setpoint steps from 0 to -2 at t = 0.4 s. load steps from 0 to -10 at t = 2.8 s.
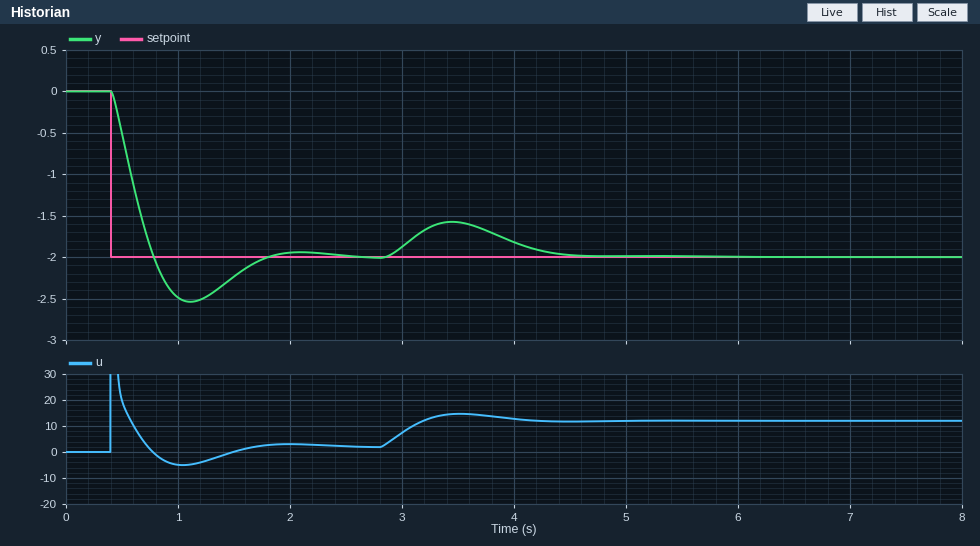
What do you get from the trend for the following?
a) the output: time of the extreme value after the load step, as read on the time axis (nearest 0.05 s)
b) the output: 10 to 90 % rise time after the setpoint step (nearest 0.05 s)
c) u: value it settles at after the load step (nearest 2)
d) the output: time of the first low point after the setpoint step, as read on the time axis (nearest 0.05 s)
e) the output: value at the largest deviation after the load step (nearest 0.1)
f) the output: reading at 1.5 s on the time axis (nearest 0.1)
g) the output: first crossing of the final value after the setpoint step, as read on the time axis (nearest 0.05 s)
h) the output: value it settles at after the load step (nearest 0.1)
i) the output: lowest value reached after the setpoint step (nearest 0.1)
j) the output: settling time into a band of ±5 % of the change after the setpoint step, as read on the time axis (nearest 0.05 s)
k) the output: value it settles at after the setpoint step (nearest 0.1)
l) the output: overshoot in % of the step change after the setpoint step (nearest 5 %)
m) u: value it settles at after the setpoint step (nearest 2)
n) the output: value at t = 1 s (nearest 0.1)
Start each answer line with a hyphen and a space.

- 3.45 s
- 0.30 s
- 12
- 1.10 s
- -1.6
- -2.2
- 0.80 s
- -2.0
- -2.5
- 1.65 s
- -2.0
- 25 %
- 2
- -2.5
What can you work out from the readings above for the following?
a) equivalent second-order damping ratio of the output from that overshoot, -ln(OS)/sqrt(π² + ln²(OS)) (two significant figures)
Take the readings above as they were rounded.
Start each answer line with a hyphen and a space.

- 0.40
